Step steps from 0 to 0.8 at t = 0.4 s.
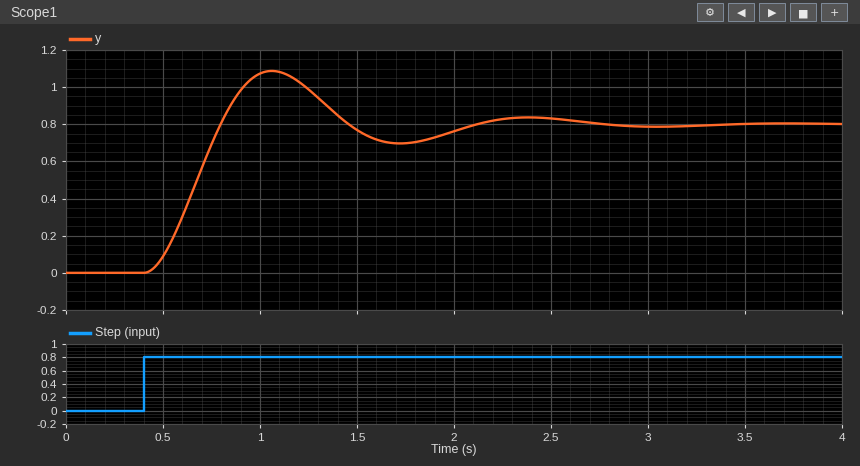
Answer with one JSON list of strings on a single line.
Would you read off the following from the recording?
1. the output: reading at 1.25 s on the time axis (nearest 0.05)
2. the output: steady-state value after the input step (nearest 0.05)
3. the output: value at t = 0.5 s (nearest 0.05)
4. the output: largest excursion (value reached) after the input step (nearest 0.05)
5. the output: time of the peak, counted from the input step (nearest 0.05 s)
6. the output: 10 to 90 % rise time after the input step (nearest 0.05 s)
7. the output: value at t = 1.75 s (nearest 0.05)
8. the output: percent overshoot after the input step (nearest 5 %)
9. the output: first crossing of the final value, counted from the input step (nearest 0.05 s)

["1.00", "0.80", "0.10", "1.10", "0.65 s", "0.25 s", "0.70", "35 %", "0.40 s"]
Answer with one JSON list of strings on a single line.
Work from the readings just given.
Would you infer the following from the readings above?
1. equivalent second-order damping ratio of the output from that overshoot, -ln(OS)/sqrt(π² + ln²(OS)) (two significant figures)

["0.32"]
